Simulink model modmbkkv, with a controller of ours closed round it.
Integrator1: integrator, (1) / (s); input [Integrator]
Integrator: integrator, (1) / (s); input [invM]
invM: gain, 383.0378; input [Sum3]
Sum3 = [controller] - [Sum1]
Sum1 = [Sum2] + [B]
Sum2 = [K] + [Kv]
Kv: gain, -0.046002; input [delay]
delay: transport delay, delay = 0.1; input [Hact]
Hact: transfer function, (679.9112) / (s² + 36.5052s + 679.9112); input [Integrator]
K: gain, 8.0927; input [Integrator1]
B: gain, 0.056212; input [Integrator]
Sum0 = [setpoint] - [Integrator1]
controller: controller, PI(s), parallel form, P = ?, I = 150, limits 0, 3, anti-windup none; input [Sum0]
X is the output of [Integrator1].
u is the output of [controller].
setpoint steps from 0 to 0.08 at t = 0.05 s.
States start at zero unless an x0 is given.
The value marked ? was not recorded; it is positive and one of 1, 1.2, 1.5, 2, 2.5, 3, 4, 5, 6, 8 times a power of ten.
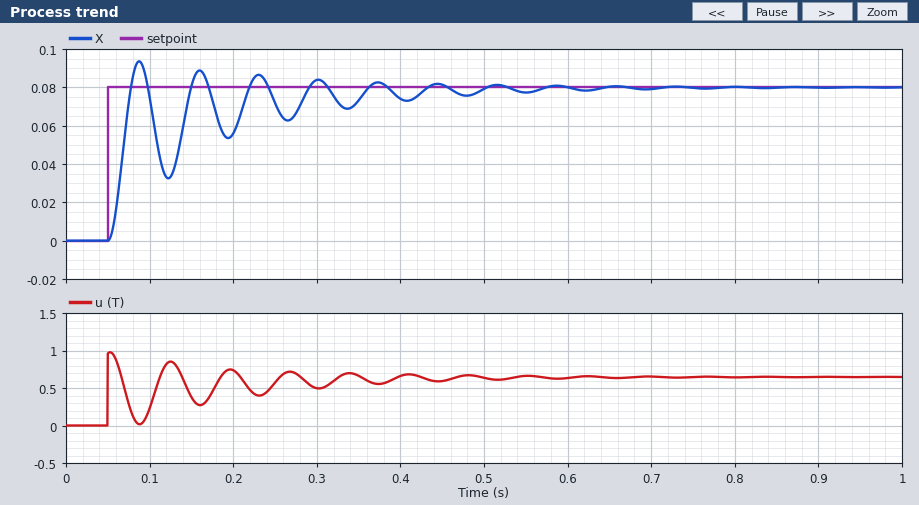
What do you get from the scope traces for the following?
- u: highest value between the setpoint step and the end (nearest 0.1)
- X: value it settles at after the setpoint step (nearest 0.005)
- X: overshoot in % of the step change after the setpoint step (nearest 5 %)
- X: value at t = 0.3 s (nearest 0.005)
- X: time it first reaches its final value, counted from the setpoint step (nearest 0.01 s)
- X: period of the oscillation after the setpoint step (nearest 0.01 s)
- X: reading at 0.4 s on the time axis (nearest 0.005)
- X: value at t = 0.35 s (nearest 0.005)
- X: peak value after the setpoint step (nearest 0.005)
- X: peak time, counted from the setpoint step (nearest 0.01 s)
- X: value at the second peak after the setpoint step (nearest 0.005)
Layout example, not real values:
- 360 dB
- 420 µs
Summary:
- 1.0
- 0.080
- 15 %
- 0.085
- 0.03 s
- 0.07 s
- 0.075
- 0.075
- 0.095
- 0.04 s
- 0.090
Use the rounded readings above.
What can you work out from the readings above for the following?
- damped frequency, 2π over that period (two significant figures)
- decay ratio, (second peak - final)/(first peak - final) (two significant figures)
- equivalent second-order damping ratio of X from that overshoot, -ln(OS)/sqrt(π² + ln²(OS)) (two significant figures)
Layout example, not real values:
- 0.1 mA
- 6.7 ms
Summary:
- 90 rad/s
- 0.67
- 0.52
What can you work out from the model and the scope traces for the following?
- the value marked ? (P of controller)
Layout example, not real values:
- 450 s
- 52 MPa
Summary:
- 12
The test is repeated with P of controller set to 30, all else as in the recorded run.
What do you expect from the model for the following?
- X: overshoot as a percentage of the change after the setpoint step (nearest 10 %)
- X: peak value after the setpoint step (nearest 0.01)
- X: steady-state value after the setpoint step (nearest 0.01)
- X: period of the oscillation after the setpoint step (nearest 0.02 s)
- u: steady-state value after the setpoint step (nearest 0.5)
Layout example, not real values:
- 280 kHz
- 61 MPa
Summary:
- 60 %
- 0.13
- 0.08
- 0.06 s
- 0.5
